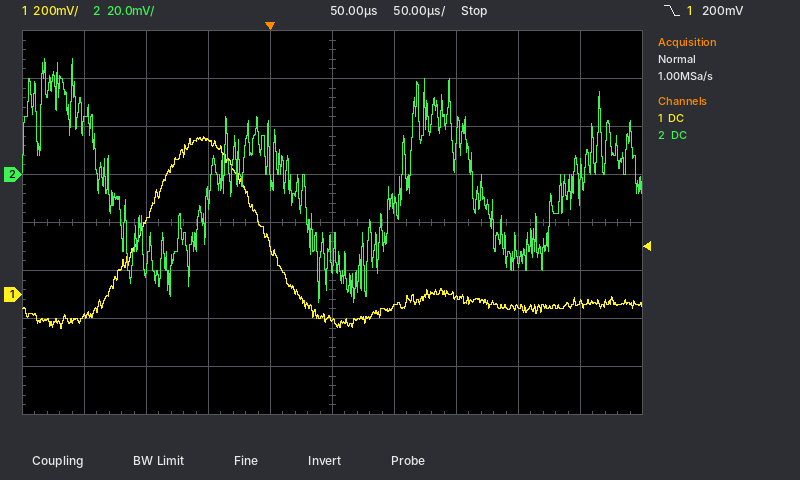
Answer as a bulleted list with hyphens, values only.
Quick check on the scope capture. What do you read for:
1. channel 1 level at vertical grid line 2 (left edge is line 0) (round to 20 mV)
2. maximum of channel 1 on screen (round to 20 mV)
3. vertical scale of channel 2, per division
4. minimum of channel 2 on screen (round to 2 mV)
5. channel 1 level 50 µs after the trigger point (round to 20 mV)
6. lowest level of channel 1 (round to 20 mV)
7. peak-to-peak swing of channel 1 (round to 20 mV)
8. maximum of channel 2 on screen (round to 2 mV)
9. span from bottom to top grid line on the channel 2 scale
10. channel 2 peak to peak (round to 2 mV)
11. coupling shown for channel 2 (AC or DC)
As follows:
- 300 mV
- 660 mV
- 20 mV
- -54 mV
- -100 mV
- -140 mV
- 800 mV
- 48 mV
- 160 mV
- 102 mV
- DC
